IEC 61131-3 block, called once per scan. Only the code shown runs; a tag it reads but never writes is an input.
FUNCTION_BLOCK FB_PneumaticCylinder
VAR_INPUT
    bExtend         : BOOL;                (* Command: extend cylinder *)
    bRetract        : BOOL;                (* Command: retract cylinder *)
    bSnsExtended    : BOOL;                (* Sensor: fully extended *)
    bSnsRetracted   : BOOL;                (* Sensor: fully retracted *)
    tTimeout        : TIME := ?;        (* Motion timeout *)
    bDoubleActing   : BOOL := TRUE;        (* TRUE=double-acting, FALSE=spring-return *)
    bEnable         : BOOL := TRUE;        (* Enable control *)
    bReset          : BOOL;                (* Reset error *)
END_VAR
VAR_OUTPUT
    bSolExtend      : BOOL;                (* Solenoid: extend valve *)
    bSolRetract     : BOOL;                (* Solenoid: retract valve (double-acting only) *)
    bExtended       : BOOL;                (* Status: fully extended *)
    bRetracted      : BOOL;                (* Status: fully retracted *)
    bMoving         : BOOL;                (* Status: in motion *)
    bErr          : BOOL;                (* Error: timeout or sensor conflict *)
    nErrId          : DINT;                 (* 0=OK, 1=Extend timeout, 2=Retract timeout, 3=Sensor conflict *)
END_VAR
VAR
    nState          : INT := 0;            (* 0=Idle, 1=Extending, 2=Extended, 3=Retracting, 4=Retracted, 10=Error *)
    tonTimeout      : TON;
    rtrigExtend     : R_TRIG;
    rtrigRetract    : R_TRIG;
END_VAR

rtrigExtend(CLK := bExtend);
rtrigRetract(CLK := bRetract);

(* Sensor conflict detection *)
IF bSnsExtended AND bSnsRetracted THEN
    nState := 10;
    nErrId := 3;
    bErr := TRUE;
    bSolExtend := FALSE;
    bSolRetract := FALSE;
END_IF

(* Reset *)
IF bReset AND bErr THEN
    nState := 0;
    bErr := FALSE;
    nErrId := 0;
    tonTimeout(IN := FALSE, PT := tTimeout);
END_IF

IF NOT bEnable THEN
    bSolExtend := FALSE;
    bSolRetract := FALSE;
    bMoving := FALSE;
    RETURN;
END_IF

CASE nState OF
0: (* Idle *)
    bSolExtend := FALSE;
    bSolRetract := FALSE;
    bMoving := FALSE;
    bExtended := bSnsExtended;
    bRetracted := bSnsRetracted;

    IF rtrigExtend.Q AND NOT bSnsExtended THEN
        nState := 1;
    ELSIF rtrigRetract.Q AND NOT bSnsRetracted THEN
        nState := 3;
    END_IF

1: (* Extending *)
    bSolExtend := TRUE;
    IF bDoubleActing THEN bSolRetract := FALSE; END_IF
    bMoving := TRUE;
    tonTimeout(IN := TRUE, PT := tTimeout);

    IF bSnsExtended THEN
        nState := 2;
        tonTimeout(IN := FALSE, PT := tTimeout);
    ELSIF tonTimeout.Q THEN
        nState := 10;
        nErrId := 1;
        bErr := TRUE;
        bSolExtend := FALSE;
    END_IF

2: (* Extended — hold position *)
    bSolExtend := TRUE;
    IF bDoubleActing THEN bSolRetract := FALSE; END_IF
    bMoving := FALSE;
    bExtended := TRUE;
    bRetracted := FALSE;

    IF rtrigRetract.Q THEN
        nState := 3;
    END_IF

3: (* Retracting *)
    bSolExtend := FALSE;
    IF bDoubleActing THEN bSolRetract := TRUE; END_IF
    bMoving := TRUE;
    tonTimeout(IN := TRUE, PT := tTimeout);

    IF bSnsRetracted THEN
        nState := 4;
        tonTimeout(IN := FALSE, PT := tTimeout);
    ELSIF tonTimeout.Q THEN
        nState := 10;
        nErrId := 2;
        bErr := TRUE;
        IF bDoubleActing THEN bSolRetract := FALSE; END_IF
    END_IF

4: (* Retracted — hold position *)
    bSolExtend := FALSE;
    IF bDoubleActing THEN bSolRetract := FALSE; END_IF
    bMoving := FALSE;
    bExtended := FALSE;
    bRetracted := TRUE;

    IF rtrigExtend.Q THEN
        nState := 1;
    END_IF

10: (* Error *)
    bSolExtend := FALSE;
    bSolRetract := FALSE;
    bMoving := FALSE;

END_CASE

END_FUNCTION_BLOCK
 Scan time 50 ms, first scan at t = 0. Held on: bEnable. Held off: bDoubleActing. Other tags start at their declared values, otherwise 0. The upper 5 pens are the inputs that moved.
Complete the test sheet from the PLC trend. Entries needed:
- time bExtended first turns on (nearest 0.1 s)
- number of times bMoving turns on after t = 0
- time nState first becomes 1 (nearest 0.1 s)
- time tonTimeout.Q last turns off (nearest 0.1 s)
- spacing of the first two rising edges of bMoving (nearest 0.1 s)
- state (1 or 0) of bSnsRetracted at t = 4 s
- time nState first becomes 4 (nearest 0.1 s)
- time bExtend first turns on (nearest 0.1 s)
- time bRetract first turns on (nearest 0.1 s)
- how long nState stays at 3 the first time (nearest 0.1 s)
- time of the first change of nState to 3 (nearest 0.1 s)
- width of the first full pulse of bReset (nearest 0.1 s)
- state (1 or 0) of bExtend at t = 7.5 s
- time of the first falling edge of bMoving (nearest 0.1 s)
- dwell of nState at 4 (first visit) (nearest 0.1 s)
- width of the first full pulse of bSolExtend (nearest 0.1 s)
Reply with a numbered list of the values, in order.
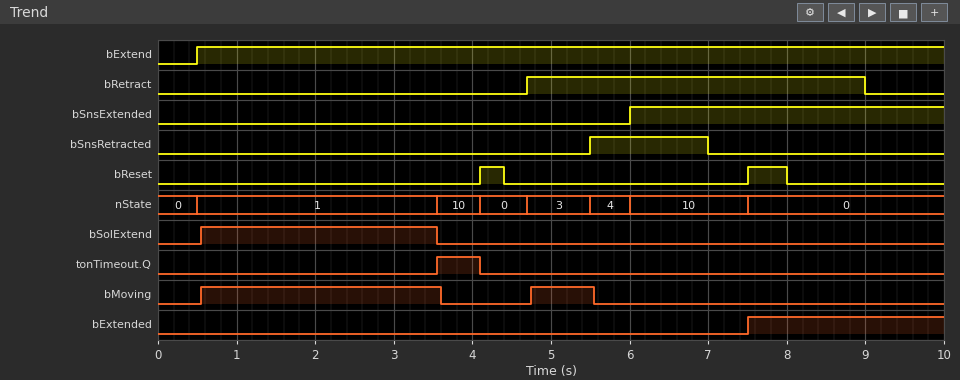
1. 7.5 s
2. 2
3. 0.5 s
4. 4.1 s
5. 4.2 s
6. 0
7. 5.5 s
8. 0.5 s
9. 4.7 s
10. 0.8 s
11. 4.7 s
12. 0.3 s
13. 1
14. 3.6 s
15. 0.5 s
16. 3.0 s
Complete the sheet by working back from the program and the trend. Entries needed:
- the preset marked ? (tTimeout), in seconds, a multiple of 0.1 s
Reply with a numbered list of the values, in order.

1. 3.0 s
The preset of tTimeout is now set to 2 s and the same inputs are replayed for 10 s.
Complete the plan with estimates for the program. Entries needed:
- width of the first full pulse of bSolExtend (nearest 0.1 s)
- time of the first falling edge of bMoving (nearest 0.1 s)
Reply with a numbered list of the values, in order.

1. 2.0 s
2. 2.6 s
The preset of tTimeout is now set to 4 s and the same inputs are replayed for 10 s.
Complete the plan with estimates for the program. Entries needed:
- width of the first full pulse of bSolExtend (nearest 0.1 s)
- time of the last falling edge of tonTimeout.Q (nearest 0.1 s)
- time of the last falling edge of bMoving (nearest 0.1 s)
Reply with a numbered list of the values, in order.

1. 4.0 s
2. 7.5 s
3. 4.6 s
